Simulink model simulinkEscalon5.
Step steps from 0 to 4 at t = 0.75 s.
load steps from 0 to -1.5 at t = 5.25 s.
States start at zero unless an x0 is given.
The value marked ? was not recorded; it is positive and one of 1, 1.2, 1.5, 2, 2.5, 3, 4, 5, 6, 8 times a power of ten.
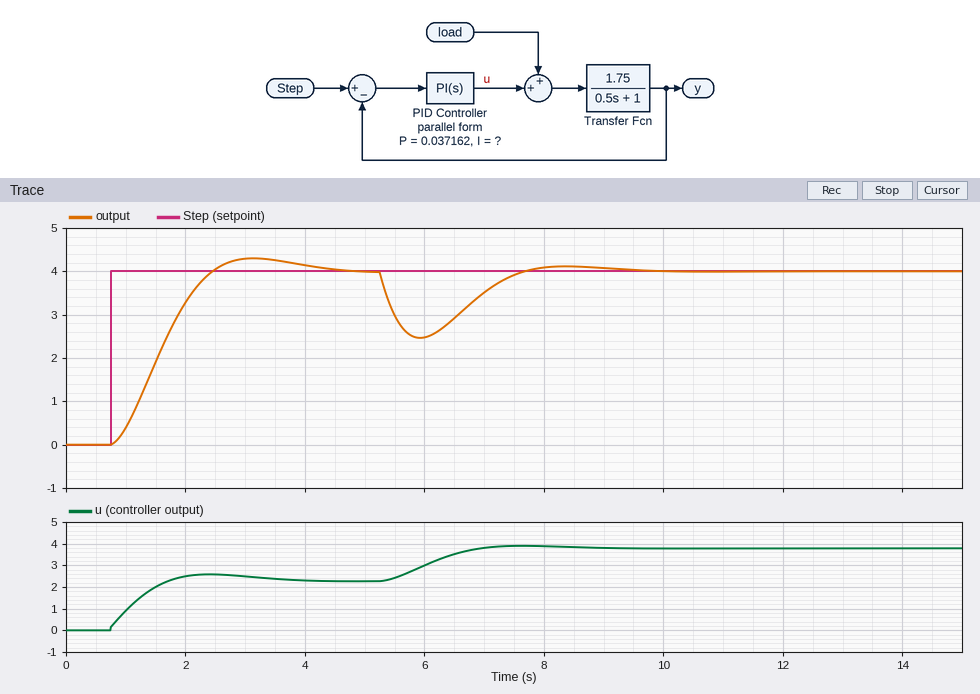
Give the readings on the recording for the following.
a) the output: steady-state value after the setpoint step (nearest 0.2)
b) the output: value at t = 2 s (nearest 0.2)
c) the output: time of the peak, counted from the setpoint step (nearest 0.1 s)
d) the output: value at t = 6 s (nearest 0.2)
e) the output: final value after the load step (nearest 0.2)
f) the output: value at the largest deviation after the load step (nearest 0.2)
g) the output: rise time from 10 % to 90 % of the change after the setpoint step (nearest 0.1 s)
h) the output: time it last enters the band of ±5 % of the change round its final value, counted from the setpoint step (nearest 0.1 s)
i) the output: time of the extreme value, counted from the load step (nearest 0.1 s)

4.0
3.2
2.4 s
2.4
4.0
2.4
1.2 s
3.0 s
0.7 s
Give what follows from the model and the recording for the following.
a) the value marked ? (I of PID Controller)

0.8
